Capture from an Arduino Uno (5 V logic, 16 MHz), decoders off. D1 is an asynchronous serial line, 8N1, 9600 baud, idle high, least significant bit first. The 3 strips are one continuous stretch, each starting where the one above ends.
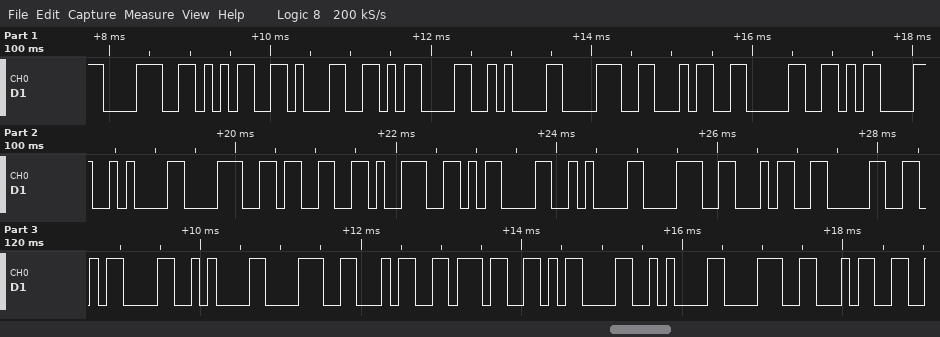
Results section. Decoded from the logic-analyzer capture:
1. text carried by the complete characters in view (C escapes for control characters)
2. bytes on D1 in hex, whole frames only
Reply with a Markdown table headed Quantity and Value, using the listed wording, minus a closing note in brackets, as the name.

| Quantity | Value |
|---|---|
| text carried by the complete characters in view | "851\r\n840\r\n839\r\n840\r\n847\r\n84" |
| bytes on D1 in hex, whole frames only | 38 35 31 0D 0A 38 34 30 0D 0A 38 33 39 0D 0A 38 34 30 0D 0A 38 34 37 0D 0A 38 34 |
